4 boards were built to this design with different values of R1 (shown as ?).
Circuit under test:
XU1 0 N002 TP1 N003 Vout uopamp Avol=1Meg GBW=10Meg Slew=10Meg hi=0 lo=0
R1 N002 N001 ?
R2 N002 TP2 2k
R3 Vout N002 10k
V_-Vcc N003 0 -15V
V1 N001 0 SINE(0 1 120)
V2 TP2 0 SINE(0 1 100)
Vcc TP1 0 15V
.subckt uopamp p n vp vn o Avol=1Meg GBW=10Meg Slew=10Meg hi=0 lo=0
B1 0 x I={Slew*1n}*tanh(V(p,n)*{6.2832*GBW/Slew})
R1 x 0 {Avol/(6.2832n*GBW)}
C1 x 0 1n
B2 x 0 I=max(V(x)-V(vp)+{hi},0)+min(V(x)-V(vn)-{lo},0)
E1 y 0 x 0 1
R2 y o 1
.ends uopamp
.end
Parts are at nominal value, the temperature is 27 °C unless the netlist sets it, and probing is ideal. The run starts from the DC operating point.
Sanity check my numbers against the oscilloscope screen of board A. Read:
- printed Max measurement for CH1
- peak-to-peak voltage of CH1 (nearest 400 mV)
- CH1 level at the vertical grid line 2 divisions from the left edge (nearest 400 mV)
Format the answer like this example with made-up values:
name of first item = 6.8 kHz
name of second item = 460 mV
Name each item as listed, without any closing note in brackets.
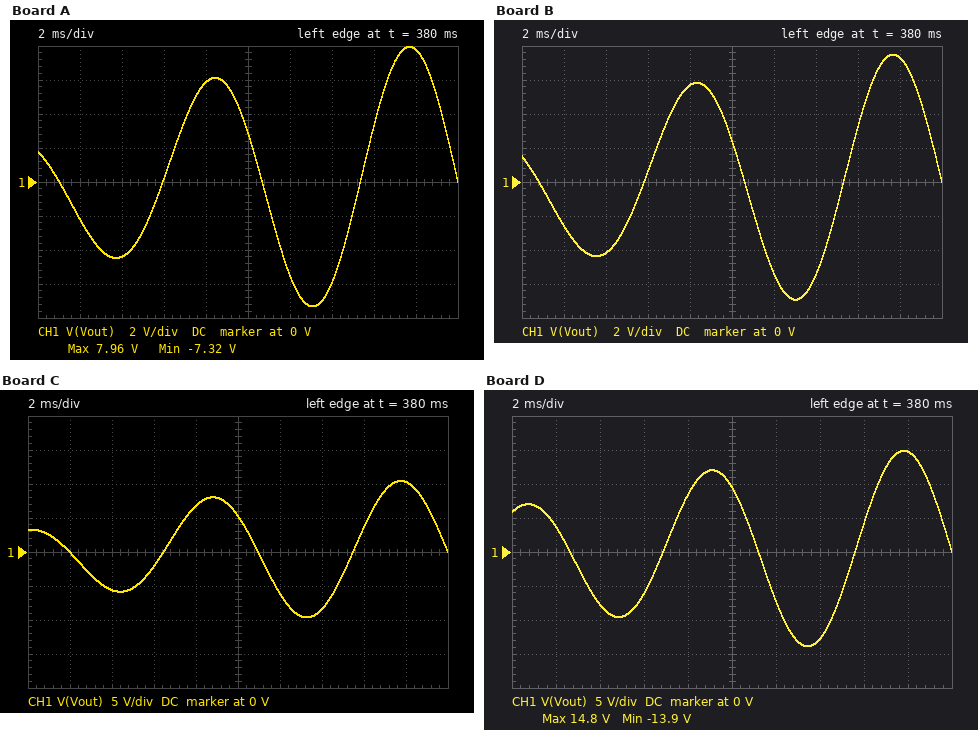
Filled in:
printed Max measurement for CH1 = 7.96 V
peak-to-peak voltage of CH1 = 15.2 V
CH1 level at the vertical grid line 2 divisions from the left edge = -4.4 V
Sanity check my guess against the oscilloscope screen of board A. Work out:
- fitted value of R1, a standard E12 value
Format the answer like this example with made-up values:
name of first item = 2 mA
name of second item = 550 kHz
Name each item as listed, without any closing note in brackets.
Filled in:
fitted value of R1, a standard E12 value = 3.3 kΩ
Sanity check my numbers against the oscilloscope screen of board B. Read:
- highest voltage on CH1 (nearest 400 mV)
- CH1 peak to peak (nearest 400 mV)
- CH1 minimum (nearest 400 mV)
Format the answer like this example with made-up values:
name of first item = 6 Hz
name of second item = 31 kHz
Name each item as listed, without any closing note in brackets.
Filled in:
highest voltage on CH1 = 7.6 V
CH1 peak to peak = 14.4 V
CH1 minimum = -6.8 V
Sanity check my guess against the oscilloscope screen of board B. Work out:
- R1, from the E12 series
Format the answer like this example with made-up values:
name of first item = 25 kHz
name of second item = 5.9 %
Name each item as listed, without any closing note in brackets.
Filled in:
R1, from the E12 series = 3.9 kΩ
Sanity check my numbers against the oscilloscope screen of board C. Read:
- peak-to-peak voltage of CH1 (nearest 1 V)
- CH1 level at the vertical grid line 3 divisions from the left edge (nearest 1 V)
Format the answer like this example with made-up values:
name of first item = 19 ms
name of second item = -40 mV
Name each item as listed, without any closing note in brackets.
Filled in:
peak-to-peak voltage of CH1 = 20 V
CH1 level at the vertical grid line 3 divisions from the left edge = -2 V
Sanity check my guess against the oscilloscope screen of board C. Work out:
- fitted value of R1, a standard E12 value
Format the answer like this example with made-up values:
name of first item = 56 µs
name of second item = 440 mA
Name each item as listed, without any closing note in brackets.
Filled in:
fitted value of R1, a standard E12 value = 1.8 kΩ
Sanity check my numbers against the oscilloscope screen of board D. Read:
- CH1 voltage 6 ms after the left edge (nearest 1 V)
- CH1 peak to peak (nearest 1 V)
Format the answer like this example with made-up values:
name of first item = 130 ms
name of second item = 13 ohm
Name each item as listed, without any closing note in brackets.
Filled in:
CH1 voltage 6 ms after the left edge = -6 V
CH1 peak to peak = 29 V
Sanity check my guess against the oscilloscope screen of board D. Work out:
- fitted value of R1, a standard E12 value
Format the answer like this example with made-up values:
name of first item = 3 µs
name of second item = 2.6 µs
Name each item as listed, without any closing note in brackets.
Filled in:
fitted value of R1, a standard E12 value = 1 kΩ
